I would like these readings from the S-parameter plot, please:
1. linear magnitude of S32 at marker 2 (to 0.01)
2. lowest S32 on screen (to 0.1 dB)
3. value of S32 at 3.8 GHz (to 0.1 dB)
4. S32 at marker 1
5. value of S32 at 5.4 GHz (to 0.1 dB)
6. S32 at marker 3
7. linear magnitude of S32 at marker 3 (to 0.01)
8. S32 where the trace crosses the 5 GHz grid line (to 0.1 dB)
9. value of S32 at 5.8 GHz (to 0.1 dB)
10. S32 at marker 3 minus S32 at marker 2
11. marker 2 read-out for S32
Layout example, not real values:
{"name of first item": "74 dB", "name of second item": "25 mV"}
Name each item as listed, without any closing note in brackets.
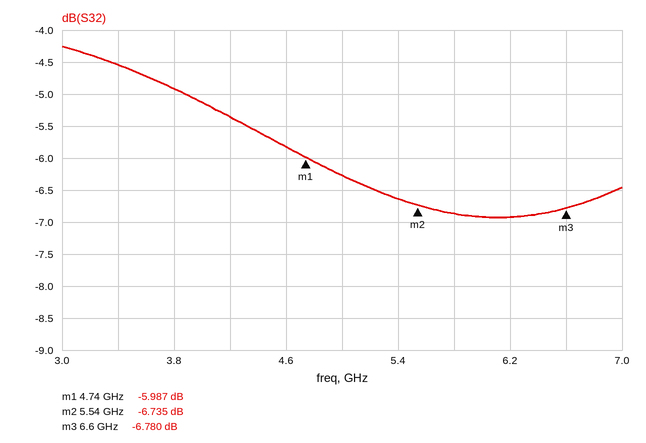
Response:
{"linear magnitude of S32 at marker 2": "0.46", "lowest S32 on screen": "-6.9 dB", "value of S32 at 3.8 GHz": "-4.9 dB", "S32 at marker 1": "-5.987 dB", "value of S32 at 5.4 GHz": "-6.6 dB", "S32 at marker 3": "-6.780 dB", "linear magnitude of S32 at marker 3": "0.46", "S32 where the trace crosses the 5 GHz grid line": "-6.3 dB", "value of S32 at 5.8 GHz": "-6.9 dB", "S32 at marker 3 minus S32 at marker 2": "-0.045 dB", "marker 2 read-out for S32": "-6.735 dB"}
